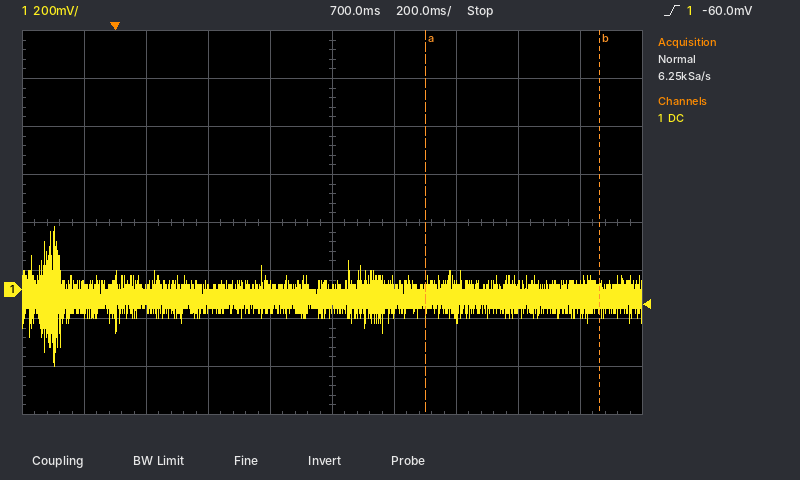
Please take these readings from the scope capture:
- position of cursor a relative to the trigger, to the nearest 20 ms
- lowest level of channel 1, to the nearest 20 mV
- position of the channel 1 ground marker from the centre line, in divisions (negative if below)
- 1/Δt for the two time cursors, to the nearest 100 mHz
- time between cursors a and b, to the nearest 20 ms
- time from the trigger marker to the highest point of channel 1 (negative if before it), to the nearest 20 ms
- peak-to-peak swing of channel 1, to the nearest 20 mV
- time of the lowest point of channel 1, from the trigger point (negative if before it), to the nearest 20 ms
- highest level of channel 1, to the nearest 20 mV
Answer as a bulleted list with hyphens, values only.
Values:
- +1.00 s
- -320 mV
- -1.4 div
- 1.8 Hz
- 560 ms
- -200 ms
- 580 mV
- -200 ms
- 260 mV
